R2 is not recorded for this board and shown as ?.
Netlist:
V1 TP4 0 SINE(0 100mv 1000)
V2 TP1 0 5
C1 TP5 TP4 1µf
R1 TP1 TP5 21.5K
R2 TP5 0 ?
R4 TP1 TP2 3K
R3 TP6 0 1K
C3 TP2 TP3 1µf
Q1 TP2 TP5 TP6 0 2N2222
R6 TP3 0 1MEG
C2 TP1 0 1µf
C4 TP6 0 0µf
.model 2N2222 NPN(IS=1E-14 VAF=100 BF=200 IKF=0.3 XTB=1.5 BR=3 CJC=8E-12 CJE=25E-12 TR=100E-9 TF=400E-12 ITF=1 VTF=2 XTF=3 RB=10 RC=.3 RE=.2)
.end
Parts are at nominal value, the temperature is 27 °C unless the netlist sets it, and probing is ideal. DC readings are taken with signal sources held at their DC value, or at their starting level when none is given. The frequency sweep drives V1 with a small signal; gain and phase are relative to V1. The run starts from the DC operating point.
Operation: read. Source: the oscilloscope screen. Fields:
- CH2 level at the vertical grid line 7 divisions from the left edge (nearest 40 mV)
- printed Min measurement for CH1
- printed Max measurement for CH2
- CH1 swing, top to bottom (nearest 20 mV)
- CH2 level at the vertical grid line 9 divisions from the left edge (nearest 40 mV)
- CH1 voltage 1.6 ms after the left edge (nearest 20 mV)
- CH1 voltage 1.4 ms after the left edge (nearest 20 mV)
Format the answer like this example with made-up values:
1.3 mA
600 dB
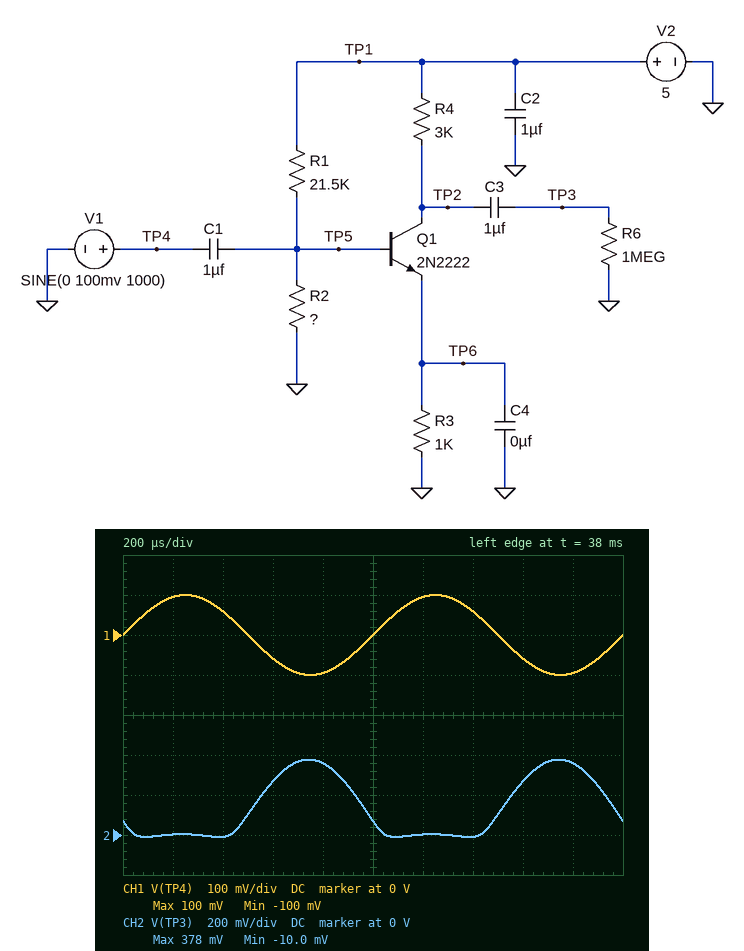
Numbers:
0 V
-100 mV
378 mV
200 mV
360 mV
-60 mV
60 mV
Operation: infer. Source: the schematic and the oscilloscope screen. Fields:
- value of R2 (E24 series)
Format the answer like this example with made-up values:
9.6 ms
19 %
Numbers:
15 kΩ
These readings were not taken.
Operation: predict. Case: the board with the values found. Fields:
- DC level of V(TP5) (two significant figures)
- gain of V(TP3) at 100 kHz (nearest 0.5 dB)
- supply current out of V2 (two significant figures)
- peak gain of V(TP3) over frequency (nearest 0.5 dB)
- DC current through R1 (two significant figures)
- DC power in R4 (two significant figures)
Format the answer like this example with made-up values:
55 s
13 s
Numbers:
1.9 V
-3.5 dB
1.4 mA
0 dB
140 µA
4.5 mW
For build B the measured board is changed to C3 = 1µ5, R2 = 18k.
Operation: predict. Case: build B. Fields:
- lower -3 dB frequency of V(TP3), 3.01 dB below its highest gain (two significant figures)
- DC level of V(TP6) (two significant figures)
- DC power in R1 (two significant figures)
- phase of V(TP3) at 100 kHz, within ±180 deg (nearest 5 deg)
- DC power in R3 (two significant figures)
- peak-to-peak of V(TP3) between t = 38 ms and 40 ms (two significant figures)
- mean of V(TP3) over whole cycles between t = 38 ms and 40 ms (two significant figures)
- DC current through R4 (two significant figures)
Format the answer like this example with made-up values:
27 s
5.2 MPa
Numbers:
670 kHz
1.3 V
440 µW
35 deg
1.6 mW
280 mV
95 mV
1.2 mA
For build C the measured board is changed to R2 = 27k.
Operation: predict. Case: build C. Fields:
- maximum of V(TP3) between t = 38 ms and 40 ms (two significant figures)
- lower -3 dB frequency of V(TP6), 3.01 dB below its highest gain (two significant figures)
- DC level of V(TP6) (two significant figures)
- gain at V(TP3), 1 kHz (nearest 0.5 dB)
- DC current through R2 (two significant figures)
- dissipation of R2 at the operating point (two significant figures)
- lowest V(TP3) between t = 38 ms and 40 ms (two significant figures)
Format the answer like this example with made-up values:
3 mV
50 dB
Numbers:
130 mV
220 Hz
1.3 V
-5.5 dB
72 µA
140 µW
-14 mV
